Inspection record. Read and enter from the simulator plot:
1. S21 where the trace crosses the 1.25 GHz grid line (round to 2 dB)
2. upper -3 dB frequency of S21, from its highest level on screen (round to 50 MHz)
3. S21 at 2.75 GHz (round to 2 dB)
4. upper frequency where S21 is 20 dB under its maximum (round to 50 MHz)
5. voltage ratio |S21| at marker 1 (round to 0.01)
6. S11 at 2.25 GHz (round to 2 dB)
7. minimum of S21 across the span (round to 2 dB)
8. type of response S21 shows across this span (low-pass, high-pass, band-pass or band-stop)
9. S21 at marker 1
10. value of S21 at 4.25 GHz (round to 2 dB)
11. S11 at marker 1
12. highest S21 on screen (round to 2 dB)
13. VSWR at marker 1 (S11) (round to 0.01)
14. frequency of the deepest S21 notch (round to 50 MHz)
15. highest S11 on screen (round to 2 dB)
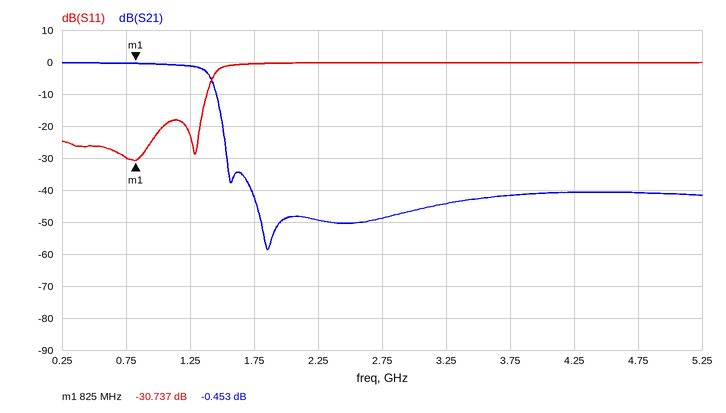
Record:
-2 dB
1.40 GHz
-48 dB
1.50 GHz
0.95
0 dB
-58 dB
low-pass
-0.453 dB
-40 dB
-30.737 dB
0 dB
1.06
1.85 GHz
0 dB
